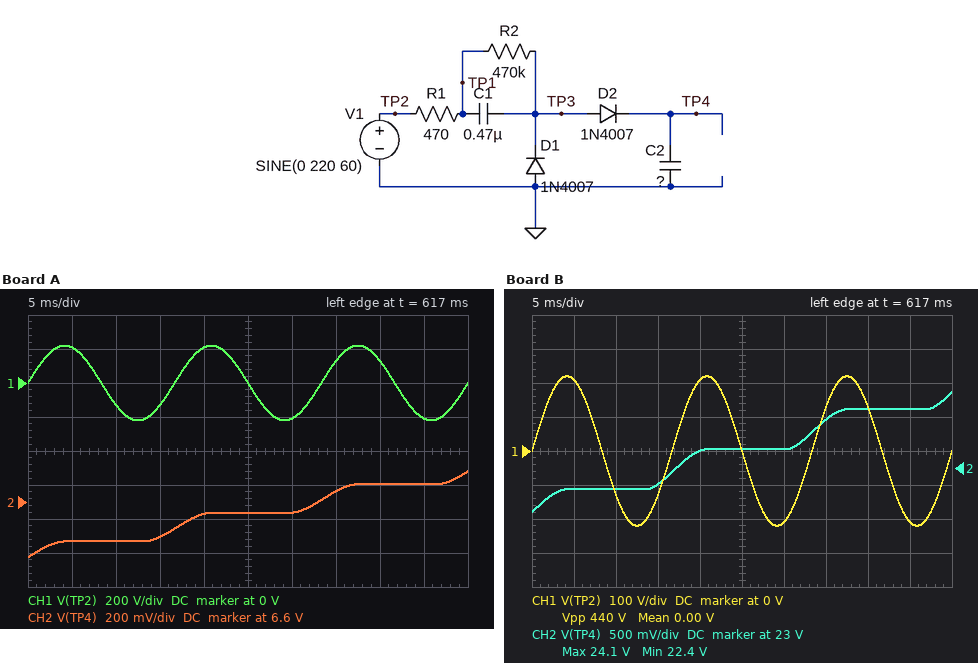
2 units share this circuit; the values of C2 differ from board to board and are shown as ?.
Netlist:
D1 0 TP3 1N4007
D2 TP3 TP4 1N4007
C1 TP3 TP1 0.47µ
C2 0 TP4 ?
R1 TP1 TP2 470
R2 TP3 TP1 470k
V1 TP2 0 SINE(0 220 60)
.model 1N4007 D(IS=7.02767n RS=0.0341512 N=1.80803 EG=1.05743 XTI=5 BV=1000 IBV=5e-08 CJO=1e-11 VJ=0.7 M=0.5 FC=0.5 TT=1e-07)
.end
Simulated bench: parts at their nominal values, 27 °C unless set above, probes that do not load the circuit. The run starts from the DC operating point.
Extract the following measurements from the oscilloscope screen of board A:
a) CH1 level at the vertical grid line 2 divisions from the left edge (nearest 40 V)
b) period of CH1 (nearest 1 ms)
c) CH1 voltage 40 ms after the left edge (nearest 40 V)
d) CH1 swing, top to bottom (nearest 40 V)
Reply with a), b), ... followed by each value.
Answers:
a) -120 V
b) 17 ms
c) 120 V
d) 440 V
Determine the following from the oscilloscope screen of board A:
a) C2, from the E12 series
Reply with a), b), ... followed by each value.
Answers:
a) 1.2 mF
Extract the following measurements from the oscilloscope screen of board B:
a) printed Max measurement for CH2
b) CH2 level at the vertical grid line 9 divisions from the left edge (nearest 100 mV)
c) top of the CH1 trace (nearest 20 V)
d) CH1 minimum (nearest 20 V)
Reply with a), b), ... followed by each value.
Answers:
a) 24.1 V
b) 23.9 V
c) 220 V
d) -220 V
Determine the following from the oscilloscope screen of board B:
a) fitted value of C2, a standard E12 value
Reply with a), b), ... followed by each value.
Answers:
a) 330 µF
